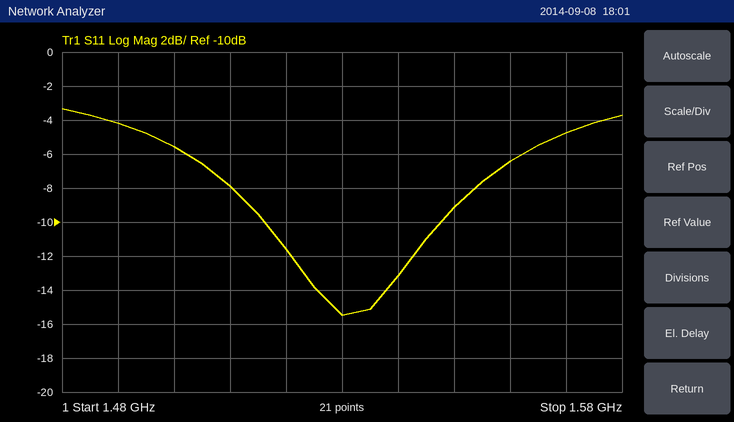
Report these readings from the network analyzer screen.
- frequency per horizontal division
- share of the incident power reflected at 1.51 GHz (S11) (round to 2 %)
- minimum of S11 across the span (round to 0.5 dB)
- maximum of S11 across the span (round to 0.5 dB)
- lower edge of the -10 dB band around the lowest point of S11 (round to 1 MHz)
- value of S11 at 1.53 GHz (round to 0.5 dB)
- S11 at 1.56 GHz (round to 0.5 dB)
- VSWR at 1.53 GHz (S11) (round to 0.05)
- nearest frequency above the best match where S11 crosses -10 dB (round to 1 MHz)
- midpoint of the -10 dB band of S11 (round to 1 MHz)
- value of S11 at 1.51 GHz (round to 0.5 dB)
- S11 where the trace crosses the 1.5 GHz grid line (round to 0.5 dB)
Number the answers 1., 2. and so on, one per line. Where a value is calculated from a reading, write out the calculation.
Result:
1. 10 MHz
2. 10^(-8/10) ≈ 16 %
3. -15.5 dB
4. -3.5 dB
5. 1.516 GHz
6. -15.5 dB
7. -6.5 dB
8. |Γ| = 10^(-15.5/20) = 0.1679; VSWR = (1 + 0.1679)/(1 − 0.1679) ≈ 1.40
9. 1.548 GHz
10. 1.532 GHz
11. -8.0 dB
12. -5.5 dB
